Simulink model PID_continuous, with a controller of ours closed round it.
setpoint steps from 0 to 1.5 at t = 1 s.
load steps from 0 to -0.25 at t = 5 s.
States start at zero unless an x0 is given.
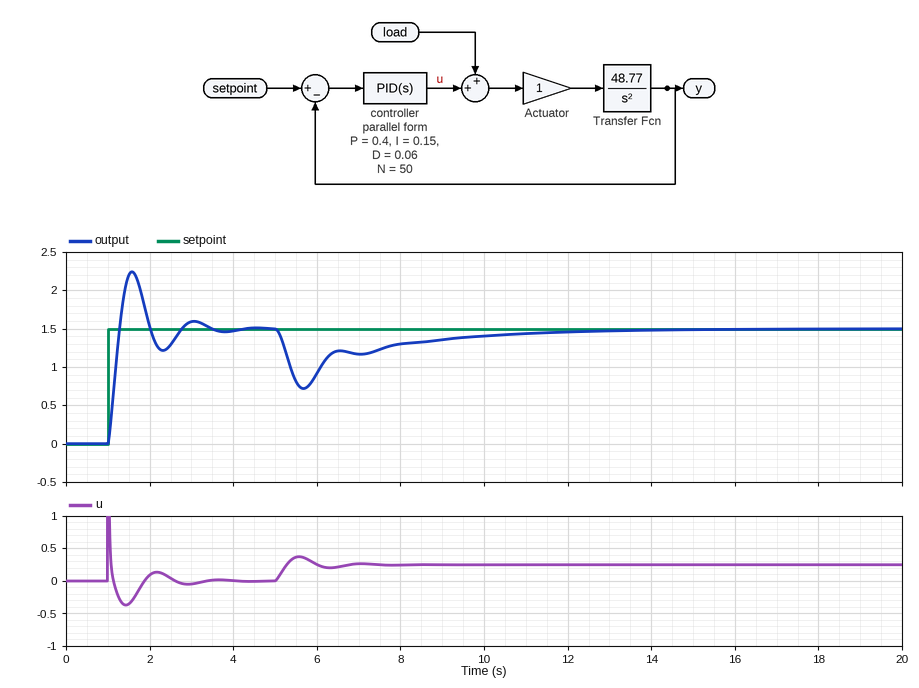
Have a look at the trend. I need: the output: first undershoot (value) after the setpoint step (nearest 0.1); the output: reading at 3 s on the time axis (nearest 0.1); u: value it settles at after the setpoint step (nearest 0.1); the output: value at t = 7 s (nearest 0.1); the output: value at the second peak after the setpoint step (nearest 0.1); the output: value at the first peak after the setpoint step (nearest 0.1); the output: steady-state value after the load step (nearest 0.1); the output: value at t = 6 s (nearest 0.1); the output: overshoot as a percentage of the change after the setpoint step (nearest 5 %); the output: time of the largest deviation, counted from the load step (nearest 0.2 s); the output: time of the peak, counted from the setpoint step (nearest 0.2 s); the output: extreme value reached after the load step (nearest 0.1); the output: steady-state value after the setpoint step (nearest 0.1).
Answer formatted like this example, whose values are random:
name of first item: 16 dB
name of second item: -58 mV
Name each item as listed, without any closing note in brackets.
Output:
the output: first undershoot (value) after the setpoint step: 1.2
the output: reading at 3 s on the time axis: 1.6
u: value it settles at after the setpoint step: 0.0
the output: value at t = 7 s: 1.2
the output: value at the second peak after the setpoint step: 1.6
the output: value at the first peak after the setpoint step: 2.2
the output: steady-state value after the load step: 1.5
the output: value at t = 6 s: 0.9
the output: overshoot as a percentage of the change after the setpoint step: 50 %
the output: time of the largest deviation, counted from the load step: 0.6 s
the output: time of the peak, counted from the setpoint step: 0.6 s
the output: extreme value reached after the load step: 0.7
the output: steady-state value after the setpoint step: 1.5
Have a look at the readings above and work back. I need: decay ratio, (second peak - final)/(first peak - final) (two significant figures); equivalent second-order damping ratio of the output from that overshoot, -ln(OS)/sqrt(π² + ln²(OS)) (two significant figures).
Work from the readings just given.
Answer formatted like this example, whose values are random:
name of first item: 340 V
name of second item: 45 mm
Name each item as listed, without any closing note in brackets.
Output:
decay ratio, (second peak - final)/(first peak - final): 0.14
equivalent second-order damping ratio of the output from that overshoot, -ln(OS)/sqrt(π² + ln²(OS)): 0.22
